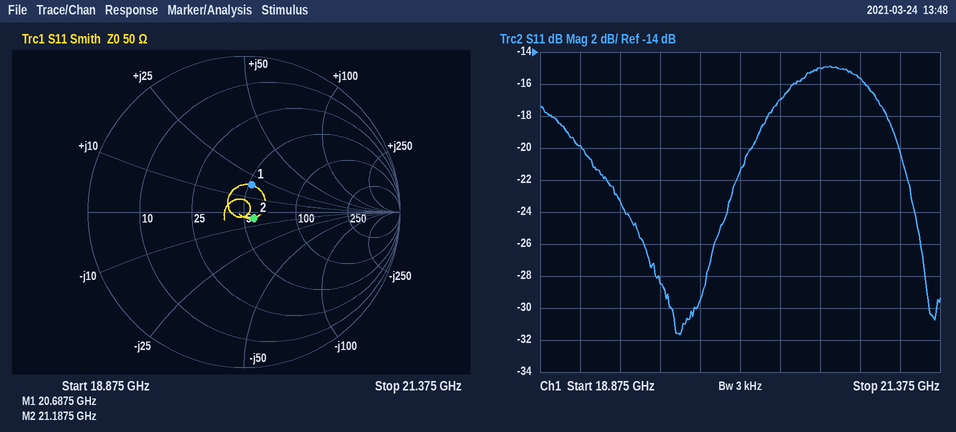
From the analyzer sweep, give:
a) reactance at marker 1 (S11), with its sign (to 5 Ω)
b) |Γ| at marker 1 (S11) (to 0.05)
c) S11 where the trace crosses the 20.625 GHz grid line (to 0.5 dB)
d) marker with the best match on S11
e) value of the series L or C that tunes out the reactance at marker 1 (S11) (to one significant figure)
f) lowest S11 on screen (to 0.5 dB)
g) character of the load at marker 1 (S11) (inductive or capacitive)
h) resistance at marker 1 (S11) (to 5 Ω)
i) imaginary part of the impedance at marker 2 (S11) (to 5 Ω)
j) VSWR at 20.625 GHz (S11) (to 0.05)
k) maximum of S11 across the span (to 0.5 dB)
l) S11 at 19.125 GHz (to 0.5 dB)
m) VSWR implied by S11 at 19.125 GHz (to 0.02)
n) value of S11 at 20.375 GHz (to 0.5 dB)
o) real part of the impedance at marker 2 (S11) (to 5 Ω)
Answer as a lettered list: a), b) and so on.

a) +20 Ω
b) 0.20
c) -15.0 dB
d) marker 2
e) 400 fF
f) -31.5 dB
g) inductive
h) 50 Ω
i) -5 Ω
j) 1.45
k) -15.0 dB
l) -20.0 dB
m) 1.22
n) -17.0 dB
o) 55 Ω
